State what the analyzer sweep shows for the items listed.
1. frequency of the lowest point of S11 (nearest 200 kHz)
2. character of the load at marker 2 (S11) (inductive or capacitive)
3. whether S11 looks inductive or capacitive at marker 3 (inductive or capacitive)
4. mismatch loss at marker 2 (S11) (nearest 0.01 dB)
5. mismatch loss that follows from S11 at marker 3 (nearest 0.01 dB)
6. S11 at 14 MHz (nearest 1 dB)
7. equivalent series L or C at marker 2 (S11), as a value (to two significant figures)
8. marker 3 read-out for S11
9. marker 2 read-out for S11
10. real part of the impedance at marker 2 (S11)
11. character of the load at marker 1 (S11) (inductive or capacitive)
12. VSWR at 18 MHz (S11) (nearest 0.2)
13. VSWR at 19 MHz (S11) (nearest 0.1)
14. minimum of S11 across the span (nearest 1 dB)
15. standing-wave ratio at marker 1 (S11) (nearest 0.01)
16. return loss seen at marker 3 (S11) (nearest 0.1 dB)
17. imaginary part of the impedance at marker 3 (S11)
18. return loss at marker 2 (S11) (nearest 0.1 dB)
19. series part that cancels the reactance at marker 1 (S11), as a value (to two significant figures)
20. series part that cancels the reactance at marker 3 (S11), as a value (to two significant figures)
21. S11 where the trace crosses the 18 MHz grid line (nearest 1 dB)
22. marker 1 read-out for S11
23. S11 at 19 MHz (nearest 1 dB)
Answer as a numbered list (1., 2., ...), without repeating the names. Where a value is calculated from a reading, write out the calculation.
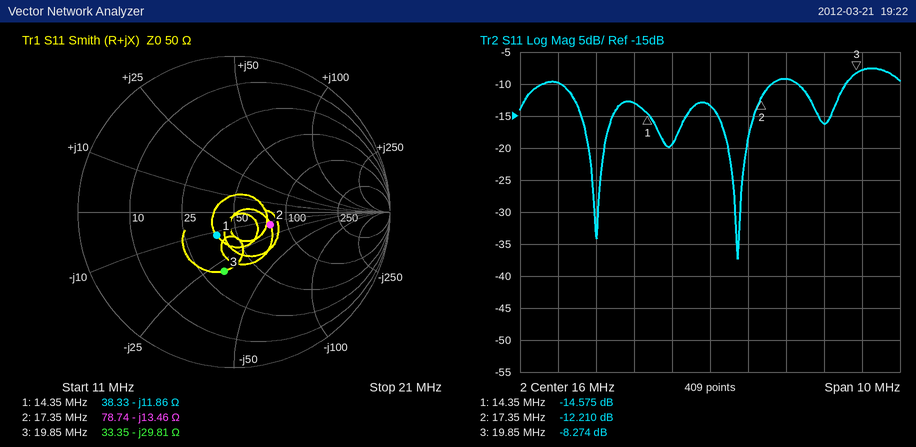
1. 16.8 MHz
2. capacitive
3. capacitive
4. −10 log10(1 − 10^(-12.21/10)) ≈ 0.27 dB
5. −10 log10(1 − 10^(-8.274/10)) ≈ 0.70 dB
6. -13 dB
7. C = 1/(2π × 17.35 MHz × 13.46 Ω) ≈ 682 pF, so 680 pF to two significant figures
8. -8.274 dB
9. -12.210 dB
10. 78.74 Ω
11. capacitive
12. |Γ| = 10^(-9/20) = 0.3548; VSWR = (1 + 0.3548)/(1 − 0.3548) ≈ 2.10, so 2.0 to the nearest 0.2
13. |Γ| = 10^(-16/20) = 0.1585; VSWR = (1 + 0.1585)/(1 − 0.1585) ≈ 1.4
14. -37 dB
15. 1.46
16. 8.3 dB
17. -29.81 Ω
18. 12.2 dB
19. L = 11.86 Ω/(2π × 14.35 MHz) ≈ 132 nH, so 130 nH to two significant figures
20. L = 29.81 Ω/(2π × 19.85 MHz) ≈ 239 nH, so 240 nH to two significant figures
21. -9 dB
22. -14.575 dB
23. -16 dB
